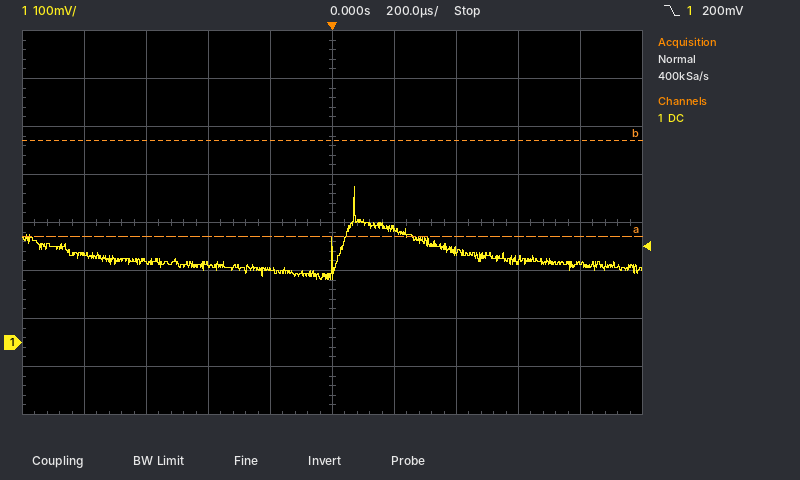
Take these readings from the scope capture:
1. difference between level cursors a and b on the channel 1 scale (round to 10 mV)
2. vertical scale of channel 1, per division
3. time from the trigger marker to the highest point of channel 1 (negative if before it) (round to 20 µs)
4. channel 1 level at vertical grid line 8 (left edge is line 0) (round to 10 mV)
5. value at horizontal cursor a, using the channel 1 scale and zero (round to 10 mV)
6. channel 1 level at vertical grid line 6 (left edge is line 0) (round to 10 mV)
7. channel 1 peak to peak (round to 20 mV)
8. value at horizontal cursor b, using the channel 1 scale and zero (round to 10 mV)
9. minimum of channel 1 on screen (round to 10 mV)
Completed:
200 mV
100 mV
+80 µs
170 mV
220 mV
240 mV
200 mV
420 mV
130 mV
